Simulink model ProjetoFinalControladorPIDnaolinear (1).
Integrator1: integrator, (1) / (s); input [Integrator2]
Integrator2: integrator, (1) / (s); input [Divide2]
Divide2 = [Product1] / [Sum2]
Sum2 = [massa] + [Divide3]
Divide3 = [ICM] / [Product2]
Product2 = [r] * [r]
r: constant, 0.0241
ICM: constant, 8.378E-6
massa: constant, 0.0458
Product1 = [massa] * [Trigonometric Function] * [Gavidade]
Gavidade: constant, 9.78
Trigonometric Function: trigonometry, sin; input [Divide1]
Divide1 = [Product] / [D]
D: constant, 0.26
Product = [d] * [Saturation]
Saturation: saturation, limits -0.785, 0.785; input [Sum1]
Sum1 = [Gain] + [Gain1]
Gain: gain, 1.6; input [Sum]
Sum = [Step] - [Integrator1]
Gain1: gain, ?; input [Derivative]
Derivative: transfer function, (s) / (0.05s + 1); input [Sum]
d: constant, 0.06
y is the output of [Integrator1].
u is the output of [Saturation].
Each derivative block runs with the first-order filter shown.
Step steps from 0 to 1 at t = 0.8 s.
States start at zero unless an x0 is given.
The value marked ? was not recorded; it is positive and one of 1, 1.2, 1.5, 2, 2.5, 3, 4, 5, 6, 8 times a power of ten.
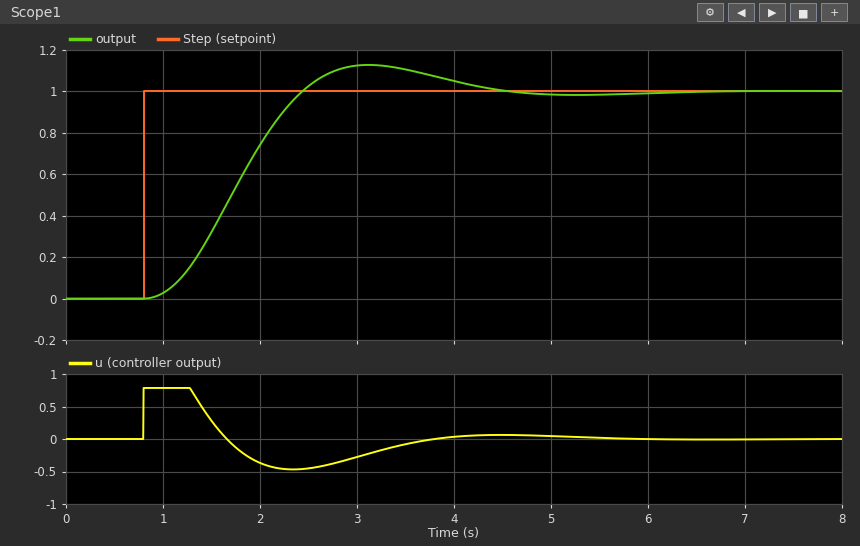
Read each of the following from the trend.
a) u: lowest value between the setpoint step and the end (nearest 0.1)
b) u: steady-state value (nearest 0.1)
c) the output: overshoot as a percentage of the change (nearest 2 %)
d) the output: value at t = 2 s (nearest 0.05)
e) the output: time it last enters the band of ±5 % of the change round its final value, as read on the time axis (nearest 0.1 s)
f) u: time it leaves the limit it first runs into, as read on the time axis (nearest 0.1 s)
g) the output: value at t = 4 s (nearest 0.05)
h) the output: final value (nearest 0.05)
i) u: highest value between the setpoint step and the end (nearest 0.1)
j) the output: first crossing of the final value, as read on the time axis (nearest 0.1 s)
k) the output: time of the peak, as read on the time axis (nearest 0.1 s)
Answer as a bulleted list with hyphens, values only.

- -0.5
- 0.0
- 12 %
- 0.75
- 4.0 s
- 1.3 s
- 1.05
- 1.00
- 0.8
- 2.4 s
- 3.1 s
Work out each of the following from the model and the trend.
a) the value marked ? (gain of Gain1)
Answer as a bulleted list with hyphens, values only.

- 1
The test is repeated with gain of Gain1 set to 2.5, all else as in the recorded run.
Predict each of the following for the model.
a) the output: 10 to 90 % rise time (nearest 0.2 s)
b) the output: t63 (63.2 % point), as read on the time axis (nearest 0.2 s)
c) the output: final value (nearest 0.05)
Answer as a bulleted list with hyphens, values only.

- 3.0 s
- 2.4 s
- 1.00
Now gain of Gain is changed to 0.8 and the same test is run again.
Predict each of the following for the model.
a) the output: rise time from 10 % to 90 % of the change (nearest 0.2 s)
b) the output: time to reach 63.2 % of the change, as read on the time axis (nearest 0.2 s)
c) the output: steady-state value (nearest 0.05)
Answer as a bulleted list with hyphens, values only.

- 1.8 s
- 2.2 s
- 1.00
